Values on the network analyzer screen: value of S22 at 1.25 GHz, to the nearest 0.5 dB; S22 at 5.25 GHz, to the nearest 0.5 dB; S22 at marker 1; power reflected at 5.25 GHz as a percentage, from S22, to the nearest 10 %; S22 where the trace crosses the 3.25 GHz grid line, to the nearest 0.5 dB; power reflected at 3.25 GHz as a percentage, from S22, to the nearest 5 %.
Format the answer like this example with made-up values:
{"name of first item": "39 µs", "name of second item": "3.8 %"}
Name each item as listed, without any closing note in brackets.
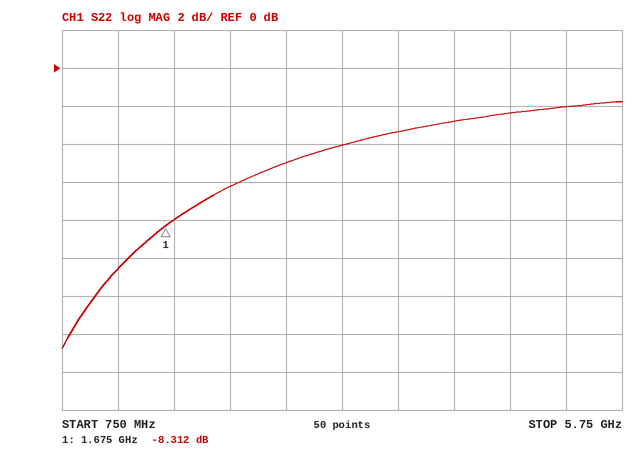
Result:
{"value of S22 at 1.25 GHz, to the nearest 0.5 dB": "-10.5 dB", "S22 at 5.25 GHz, to the nearest 0.5 dB": "-2.0 dB", "S22 at marker 1": "-8.312 dB", "power reflected at 5.25 GHz as a percentage, from S22, to the nearest 10 %": "60 %", "S22 where the trace crosses the 3.25 GHz grid line, to the nearest 0.5 dB": "-4.0 dB", "power reflected at 3.25 GHz as a percentage, from S22, to the nearest 5 %": "40 %"}
